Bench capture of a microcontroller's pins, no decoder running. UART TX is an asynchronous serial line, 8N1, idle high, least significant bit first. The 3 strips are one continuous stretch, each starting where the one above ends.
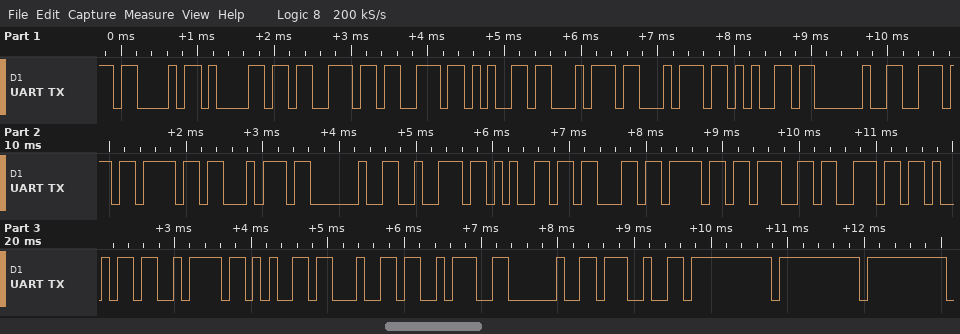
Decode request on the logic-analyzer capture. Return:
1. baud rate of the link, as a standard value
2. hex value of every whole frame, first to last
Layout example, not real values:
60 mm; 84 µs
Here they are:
9600 baud; 43 61 73 73 65 74 74 65 20 6E 6F 74 20 72 65 63 6F 67 6E 69 7A 65 64 3A 20 27 FF FF FF
